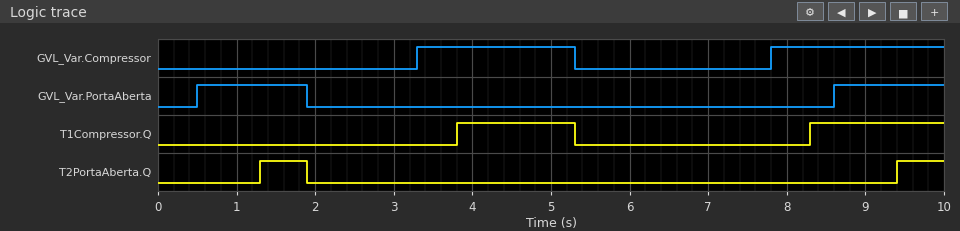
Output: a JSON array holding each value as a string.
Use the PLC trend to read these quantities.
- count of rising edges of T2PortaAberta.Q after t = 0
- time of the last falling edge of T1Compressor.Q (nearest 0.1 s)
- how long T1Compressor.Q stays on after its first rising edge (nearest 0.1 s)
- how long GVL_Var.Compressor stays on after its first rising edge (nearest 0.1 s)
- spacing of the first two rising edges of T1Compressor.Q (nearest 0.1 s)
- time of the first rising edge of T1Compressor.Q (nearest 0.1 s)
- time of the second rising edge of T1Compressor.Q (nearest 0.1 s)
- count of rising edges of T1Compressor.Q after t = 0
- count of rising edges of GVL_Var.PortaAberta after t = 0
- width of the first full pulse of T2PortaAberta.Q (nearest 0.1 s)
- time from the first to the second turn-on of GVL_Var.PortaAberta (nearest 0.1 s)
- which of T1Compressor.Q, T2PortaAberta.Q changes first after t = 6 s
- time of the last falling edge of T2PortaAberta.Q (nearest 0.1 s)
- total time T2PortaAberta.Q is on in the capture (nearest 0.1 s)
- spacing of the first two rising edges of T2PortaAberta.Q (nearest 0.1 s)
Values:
["2", "5.3 s", "1.5 s", "2.0 s", "4.5 s", "3.8 s", "8.3 s", "2", "2", "0.6 s", "8.1 s", "T1Compressor.Q", "1.9 s", "1.2 s", "8.1 s"]
